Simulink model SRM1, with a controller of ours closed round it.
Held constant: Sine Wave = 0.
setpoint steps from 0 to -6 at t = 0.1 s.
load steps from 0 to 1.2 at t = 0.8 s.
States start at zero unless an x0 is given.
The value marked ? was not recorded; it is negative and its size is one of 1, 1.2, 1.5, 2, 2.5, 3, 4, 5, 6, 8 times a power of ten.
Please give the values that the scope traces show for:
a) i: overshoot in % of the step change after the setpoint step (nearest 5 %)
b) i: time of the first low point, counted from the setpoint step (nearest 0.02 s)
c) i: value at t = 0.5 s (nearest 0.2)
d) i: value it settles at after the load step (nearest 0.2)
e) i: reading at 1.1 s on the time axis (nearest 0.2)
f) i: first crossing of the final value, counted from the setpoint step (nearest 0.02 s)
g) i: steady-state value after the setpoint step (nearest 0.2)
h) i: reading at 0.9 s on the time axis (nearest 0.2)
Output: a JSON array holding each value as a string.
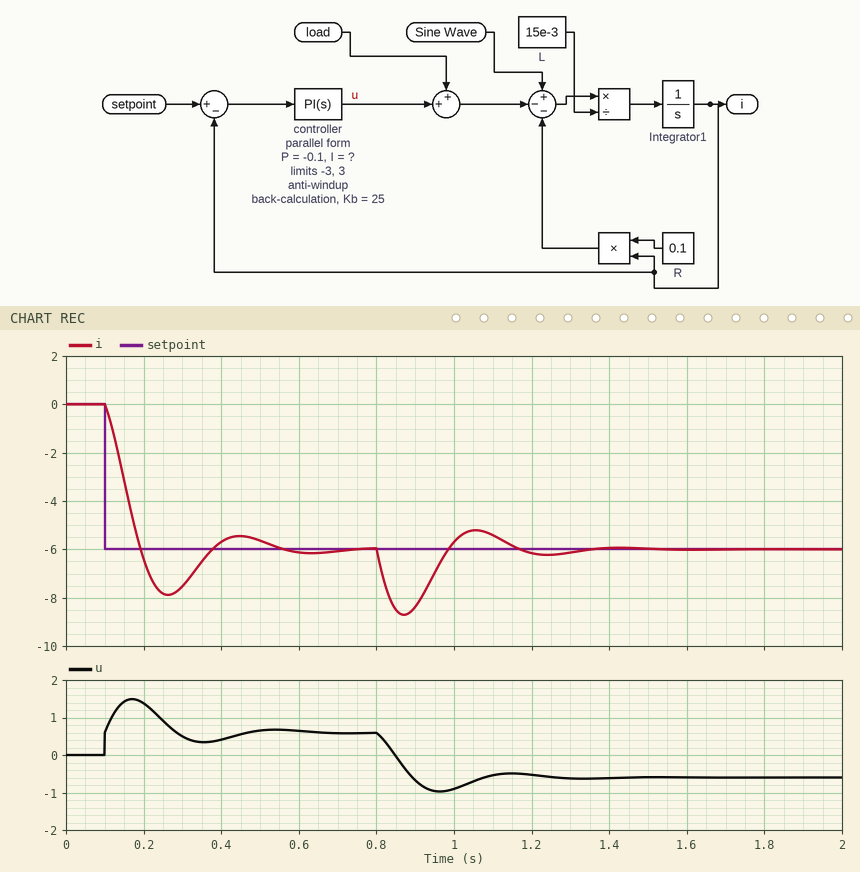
["30 %", "0.16 s", "-5.6", "-6.0", "-5.4", "0.10 s", "-6.0", "-8.4"]
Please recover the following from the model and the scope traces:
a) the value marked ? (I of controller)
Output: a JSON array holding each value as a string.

["-5"]
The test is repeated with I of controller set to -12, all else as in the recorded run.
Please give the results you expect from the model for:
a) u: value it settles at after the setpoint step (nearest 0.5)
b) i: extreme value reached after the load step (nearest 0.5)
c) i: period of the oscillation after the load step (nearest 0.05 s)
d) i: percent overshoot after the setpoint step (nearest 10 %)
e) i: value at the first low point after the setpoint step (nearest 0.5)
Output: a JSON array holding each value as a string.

["0.5", "-8.0", "0.25 s", "50 %", "-9.0"]
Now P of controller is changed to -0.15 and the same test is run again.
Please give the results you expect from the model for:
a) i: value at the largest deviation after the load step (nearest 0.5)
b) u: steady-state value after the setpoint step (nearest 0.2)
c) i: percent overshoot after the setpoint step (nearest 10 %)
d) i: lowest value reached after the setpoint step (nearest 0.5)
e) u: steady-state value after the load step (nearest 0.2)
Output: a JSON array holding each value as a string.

["-8.5", "0.6", "20 %", "-7.5", "-0.6"]
